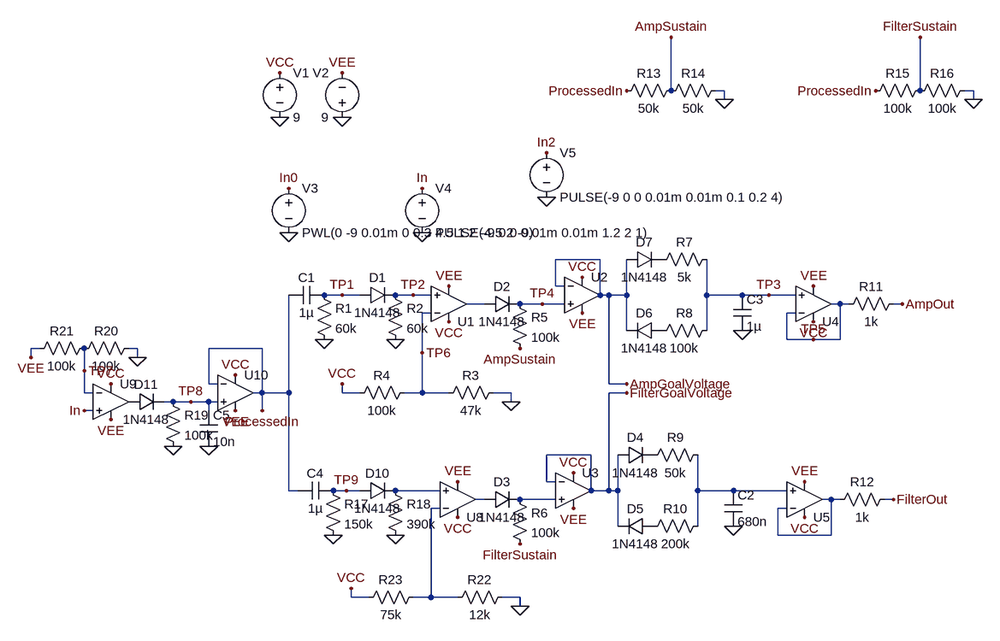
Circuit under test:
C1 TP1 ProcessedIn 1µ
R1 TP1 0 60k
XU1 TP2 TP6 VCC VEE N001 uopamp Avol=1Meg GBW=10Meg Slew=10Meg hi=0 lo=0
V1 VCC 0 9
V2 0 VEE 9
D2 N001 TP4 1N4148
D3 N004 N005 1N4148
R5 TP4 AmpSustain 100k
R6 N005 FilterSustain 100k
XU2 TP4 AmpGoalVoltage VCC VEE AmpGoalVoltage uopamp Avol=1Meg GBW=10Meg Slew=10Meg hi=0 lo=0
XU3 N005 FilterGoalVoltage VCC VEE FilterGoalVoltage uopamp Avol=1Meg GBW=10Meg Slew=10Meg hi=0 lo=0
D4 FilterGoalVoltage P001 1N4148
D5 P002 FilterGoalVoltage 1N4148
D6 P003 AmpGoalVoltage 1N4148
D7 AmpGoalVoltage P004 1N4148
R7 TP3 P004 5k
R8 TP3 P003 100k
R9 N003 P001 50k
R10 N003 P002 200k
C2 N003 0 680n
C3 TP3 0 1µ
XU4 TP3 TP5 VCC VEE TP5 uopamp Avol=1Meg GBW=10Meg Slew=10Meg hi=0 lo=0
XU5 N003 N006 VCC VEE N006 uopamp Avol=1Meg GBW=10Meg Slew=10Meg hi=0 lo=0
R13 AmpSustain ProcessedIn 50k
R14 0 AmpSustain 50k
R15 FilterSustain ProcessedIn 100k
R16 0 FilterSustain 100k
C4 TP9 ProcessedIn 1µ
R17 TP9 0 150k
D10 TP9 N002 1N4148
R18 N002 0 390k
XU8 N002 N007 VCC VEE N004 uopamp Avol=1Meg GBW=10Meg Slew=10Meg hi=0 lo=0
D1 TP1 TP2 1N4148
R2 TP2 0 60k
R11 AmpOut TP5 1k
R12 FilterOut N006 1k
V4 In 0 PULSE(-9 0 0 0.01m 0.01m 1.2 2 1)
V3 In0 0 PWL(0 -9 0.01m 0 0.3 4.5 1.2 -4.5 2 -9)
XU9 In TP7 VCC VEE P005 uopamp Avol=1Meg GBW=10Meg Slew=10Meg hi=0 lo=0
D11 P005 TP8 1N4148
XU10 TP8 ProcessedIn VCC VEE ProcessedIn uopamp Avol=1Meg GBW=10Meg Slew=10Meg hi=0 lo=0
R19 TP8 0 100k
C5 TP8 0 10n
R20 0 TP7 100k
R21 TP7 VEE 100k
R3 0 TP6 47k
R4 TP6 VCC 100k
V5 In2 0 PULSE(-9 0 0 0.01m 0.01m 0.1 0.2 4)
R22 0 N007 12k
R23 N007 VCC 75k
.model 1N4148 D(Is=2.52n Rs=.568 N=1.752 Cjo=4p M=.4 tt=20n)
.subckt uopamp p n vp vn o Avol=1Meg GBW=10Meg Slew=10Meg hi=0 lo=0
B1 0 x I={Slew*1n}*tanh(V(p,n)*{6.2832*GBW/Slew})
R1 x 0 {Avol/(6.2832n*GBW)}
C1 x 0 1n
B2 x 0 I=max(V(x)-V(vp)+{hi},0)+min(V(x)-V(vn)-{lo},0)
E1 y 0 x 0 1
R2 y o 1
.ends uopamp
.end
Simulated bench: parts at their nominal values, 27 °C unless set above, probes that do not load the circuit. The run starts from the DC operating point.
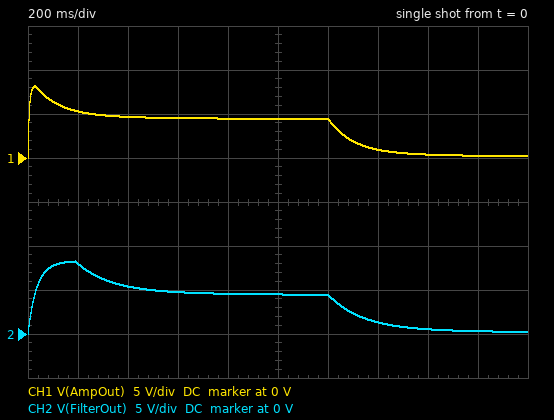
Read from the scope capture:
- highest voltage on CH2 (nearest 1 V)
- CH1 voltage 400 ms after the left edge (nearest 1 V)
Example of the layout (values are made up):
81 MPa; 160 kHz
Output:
8 V; 5 V
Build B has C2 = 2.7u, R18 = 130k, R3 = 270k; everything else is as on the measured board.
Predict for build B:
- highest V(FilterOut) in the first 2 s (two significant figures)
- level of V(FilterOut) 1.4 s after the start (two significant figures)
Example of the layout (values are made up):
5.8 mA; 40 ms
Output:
4.9 V; 3.3 V
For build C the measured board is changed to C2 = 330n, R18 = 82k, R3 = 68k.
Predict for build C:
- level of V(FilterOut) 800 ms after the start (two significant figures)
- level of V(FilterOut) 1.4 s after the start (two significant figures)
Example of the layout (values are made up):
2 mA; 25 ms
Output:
4.4 V; 510 mV
